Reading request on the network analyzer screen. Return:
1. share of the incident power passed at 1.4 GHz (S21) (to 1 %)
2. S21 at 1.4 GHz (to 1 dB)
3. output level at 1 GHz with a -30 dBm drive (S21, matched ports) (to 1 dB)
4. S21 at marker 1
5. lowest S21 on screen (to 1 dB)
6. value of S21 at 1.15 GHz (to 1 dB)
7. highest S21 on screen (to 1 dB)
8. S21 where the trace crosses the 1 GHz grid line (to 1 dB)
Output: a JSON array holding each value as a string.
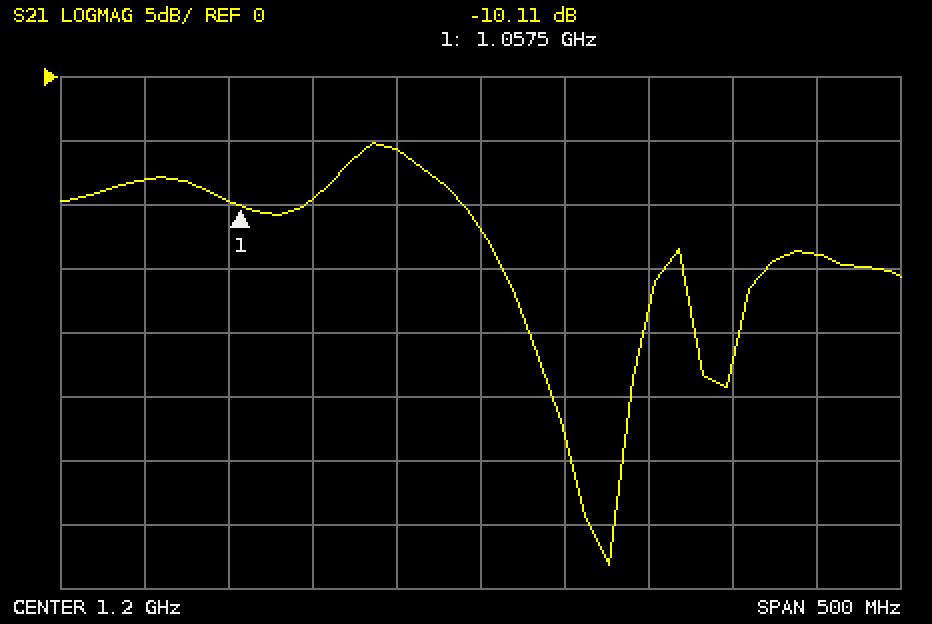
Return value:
["4 %", "-14 dB", "-38 dBm", "-10.11 dB", "-38 dB", "-6 dB", "-5 dB", "-8 dB"]
